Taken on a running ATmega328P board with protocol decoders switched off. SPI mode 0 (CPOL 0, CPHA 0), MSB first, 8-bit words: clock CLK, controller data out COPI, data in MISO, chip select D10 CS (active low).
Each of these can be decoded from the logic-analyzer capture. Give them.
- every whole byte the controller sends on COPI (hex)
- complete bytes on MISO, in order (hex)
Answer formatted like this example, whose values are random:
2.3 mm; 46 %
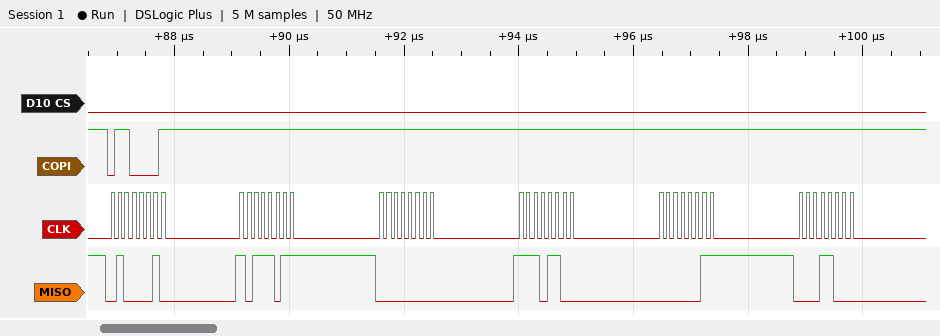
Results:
61 FF FF FF FF FF; 42 BB 00 EC 03 18
